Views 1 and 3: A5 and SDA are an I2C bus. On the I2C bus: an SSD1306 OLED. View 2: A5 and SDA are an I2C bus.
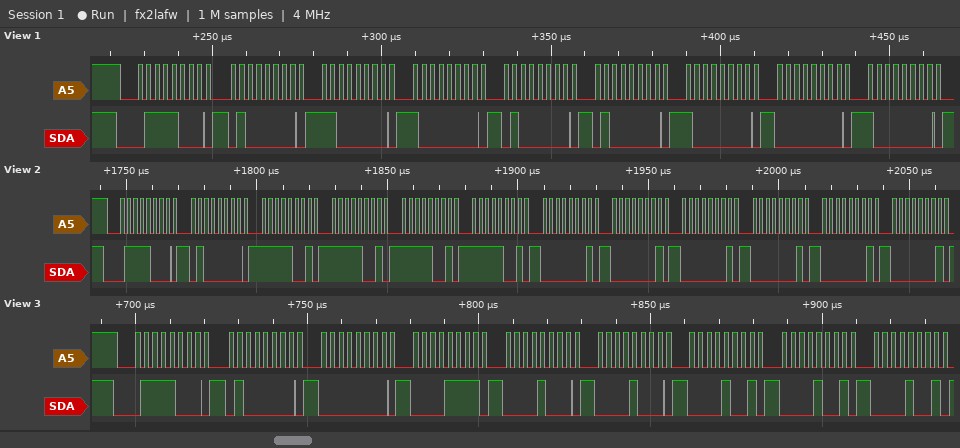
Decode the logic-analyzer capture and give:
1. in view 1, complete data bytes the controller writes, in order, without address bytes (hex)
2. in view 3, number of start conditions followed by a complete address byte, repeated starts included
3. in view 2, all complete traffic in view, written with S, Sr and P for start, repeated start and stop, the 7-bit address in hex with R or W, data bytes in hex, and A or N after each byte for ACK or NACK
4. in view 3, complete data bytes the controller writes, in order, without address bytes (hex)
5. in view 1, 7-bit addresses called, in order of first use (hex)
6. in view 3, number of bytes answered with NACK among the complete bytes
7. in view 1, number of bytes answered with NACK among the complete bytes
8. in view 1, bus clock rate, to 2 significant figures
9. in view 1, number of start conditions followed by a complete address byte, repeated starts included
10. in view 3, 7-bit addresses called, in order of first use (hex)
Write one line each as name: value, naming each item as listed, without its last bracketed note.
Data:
in view 1, complete data bytes the controller writes, in order, without address bytes: 40 C0 80 40 40 80 00 80
in view 3, number of start conditions followed by a complete address byte, repeated starts included: 1
in view 2, all complete traffic in view, written with S, Sr and P for start, repeated start and stop, the 7-bit address in hex with R or W, data bytes in hex, and A or N after each byte for ACK or NACK: S 3CW A 40 A F9 A F9 A F9 A F9 A 01 A 01 A 01 A 01 A 01 A 01 A
in view 3, complete data bytes the controller writes, in order, without address bytes: 40 00 0F 08 08 09 09 09
in view 1, 7-bit addresses called, in order of first use: 0x3C
in view 3, number of bytes answered with NACK among the complete bytes: 0
in view 1, number of bytes answered with NACK among the complete bytes: 0
in view 1, bus clock rate, to 2 significant figures: 400 kHz
in view 1, number of start conditions followed by a complete address byte, repeated starts included: 1
in view 3, 7-bit addresses called, in order of first use: 0x3C
